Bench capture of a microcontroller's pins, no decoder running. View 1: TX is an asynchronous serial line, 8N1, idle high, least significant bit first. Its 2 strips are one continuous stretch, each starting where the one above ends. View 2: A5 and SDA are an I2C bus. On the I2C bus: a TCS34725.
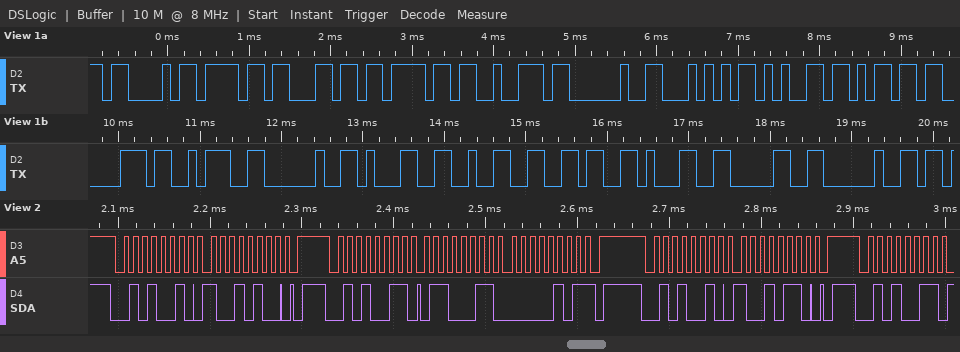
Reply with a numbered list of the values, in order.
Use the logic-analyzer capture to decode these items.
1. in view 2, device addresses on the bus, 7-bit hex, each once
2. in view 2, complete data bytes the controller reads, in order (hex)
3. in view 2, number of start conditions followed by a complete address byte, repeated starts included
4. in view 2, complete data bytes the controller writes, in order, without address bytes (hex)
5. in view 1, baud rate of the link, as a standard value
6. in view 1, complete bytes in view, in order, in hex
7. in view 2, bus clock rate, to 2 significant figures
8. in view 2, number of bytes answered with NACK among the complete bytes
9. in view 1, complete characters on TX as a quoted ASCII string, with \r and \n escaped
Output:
1. 0x29
2. 63 05
3. 4
4. 94 96
5. 9600 baud
6. 43 6F 6C 6F 72 20 54 65 6D 70 3A 20 31 32 36 31 30 20
7. 100 kHz
8. 1
9. "Color Temp: 12610 "
